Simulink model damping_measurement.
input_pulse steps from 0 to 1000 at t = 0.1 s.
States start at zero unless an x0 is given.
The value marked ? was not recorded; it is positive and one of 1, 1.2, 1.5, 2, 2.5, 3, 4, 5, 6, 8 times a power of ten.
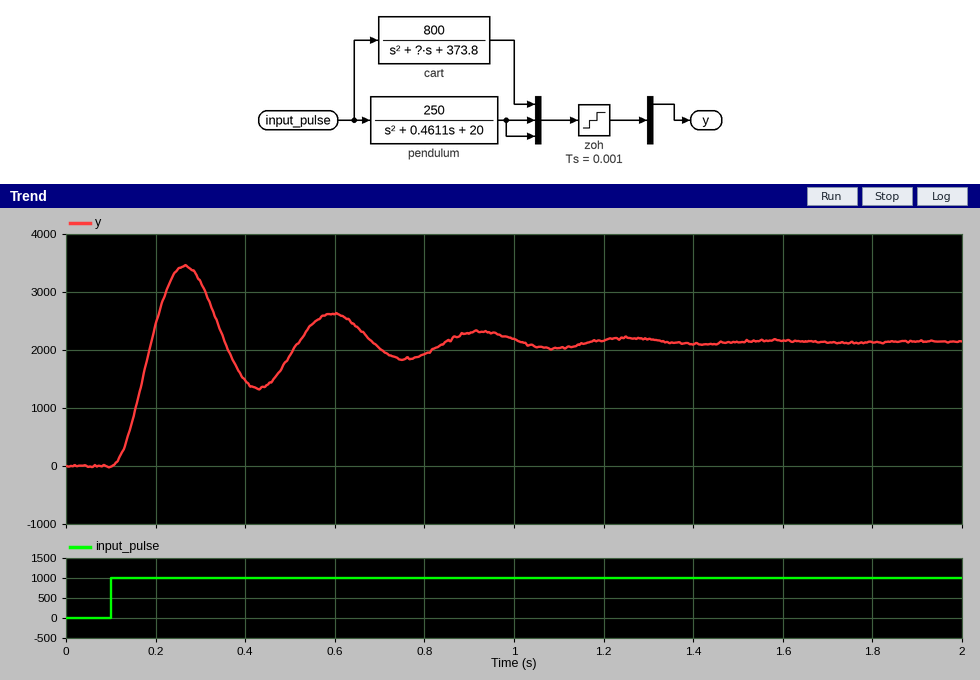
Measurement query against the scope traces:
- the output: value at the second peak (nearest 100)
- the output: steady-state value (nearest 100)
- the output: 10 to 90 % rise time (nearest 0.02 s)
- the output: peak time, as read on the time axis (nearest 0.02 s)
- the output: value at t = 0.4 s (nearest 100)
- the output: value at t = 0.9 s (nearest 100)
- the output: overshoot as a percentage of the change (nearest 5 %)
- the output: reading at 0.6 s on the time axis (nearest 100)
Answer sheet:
2600
2100
0.06 s
0.26 s
1500
2300
60 %
2600
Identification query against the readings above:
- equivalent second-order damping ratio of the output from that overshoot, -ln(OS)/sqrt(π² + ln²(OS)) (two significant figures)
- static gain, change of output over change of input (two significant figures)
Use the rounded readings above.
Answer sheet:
0.16
2.1
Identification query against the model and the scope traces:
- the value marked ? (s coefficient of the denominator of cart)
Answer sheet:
6
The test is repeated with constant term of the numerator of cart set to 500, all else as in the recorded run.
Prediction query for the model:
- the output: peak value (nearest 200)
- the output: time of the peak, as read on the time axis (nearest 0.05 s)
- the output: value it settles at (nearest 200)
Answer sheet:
2200
0.25 s
1400
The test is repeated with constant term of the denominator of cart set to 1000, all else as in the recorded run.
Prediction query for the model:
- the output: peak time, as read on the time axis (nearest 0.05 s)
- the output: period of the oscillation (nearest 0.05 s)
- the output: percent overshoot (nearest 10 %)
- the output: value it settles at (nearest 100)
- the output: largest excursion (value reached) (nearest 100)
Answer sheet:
0.20 s
0.20 s
70 %
800
1400
